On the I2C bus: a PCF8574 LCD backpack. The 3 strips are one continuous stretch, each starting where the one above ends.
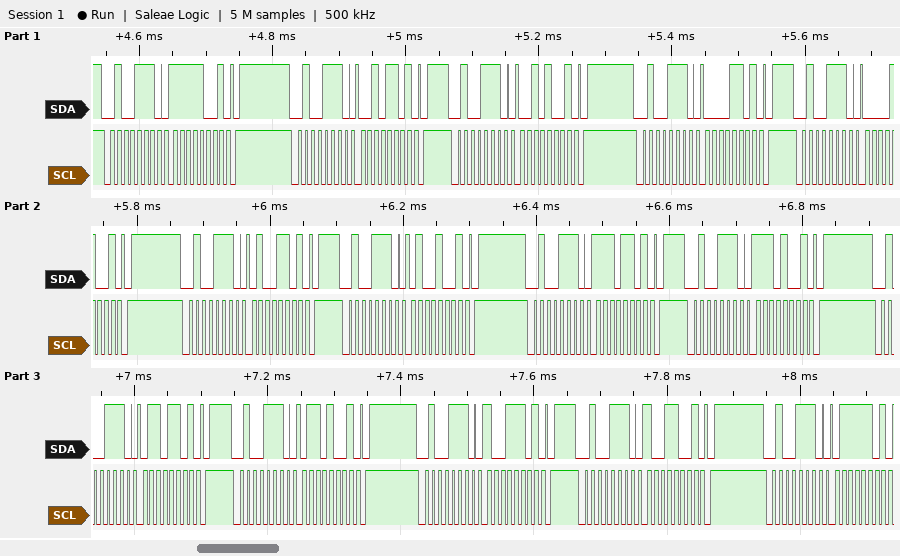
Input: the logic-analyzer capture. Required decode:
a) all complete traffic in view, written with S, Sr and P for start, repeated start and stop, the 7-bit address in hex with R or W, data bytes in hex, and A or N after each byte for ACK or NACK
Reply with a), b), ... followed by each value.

a) S 27W A F9 A P S 27W A 2D A P S 27W A 29 A P S 27W A 0D A P S 27W A 09 A P S 27W A 4D A P S 27W A 49 A P S 27W A ED A P S 27W A E9 A P S 27W A 6D A P S 27W A 69 A P S 27W A 9D A P S 27W A 99 A P S 27W A 7D A
